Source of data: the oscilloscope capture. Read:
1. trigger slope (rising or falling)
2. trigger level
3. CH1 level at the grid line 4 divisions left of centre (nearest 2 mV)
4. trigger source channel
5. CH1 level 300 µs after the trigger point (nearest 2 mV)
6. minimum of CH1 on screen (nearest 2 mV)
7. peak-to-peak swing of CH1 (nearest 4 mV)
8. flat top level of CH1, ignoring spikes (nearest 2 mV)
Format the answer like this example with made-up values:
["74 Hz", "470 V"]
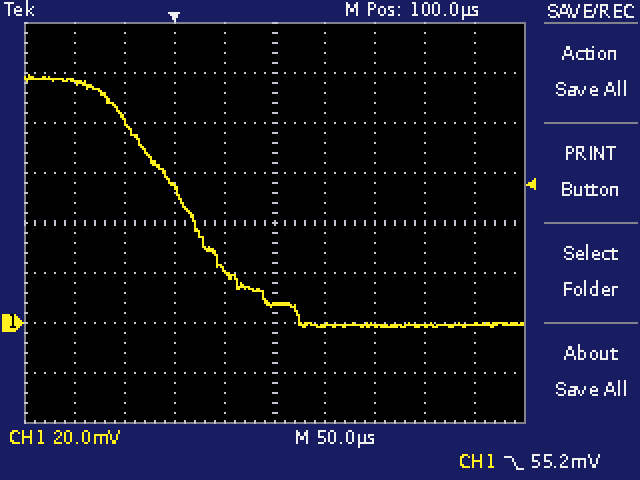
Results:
["falling", "55.2 mV", "96 mV", "CH1", "0 mV", "-2 mV", "100 mV", "98 mV"]
